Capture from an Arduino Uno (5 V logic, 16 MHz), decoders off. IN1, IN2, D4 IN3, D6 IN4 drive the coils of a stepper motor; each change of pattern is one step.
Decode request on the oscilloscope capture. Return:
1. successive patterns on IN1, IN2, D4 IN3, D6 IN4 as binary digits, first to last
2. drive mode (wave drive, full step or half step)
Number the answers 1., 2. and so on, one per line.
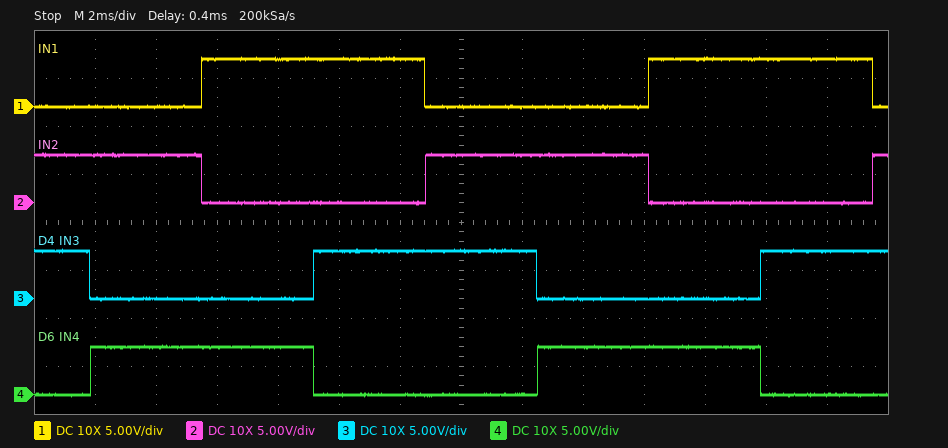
1. 0110 0101 1001 1010 0110 0101 1001 1010 0110
2. full step
